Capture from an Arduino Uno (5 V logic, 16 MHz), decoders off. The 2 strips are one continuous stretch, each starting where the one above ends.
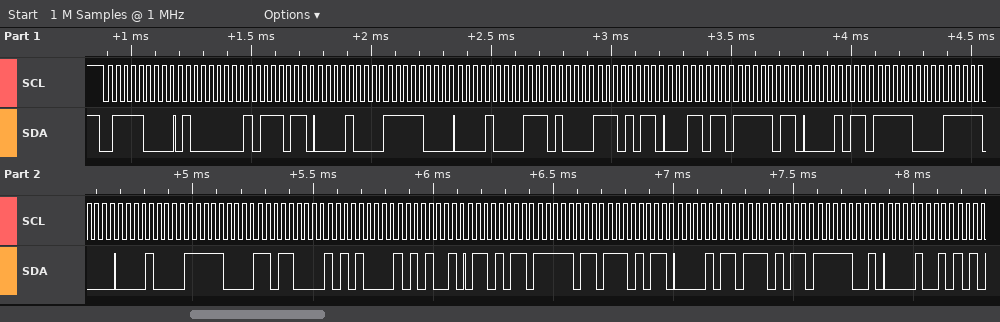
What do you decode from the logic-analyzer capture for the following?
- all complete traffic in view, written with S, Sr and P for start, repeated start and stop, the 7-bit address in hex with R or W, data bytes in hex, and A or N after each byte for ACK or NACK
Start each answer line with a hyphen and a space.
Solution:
- S 3CW A 40 A BB A 08 A F8 A 08 A E8 A EB A 1B A FB A 0B A F8 A F8 A 08 A F8 A D8 A A8 A A9 A 6B A FB A EB A 0B A EB A F9 A 09 A
